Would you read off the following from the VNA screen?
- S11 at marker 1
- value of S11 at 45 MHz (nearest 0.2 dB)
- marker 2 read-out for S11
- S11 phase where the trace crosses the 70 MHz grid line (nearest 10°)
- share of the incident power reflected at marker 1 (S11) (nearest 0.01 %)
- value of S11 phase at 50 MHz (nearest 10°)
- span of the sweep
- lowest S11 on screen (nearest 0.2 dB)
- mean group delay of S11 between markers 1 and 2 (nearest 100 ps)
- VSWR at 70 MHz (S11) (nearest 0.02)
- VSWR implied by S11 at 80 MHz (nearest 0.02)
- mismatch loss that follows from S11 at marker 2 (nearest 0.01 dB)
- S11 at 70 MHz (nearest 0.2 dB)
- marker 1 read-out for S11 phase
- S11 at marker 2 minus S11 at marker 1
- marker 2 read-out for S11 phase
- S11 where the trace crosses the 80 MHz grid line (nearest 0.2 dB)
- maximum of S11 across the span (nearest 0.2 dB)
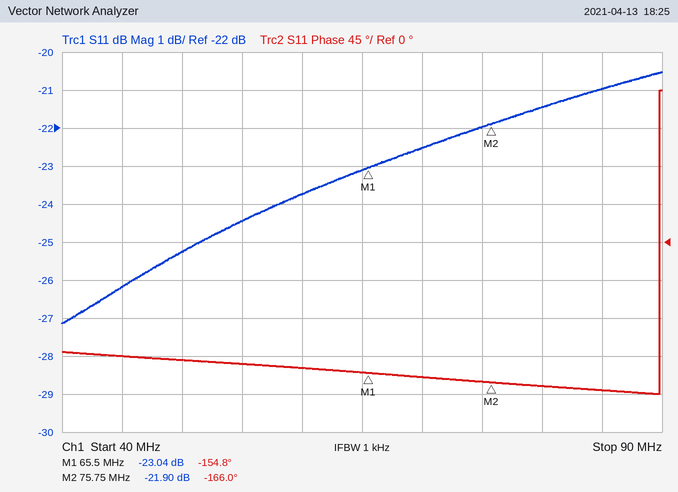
-23.04 dB
-26.2 dB
-21.90 dB
-160°
0.50 %
-140°
50 MHz
-27.2 dB
3.0 ns
1.16
1.18
0.03 dB
-22.6 dB
-154.8°
1.14 dB
-166.0°
-21.4 dB
-20.6 dB
